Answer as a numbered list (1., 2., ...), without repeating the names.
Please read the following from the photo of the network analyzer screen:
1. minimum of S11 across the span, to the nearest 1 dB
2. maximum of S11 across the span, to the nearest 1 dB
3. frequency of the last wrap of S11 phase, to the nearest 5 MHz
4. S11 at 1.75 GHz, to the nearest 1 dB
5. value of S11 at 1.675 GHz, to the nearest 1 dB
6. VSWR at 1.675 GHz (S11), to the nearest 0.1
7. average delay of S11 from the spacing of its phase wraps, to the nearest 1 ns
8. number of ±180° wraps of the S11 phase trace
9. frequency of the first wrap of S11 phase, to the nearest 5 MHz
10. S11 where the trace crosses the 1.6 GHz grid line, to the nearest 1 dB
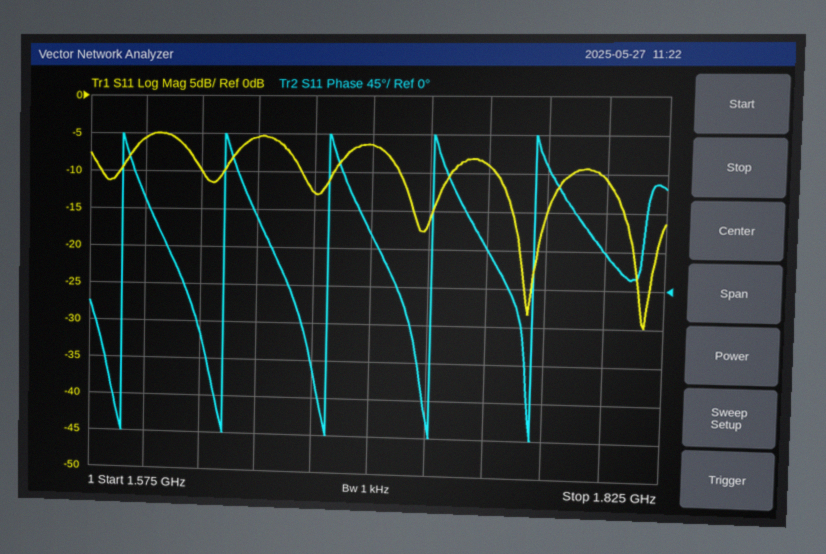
1. -30 dB
2. -5 dB
3. 1.770 GHz
4. -9 dB
5. -13 dB
6. 1.6
7. 22 ns
8. 5
9. 1.590 GHz
10. -6 dB
